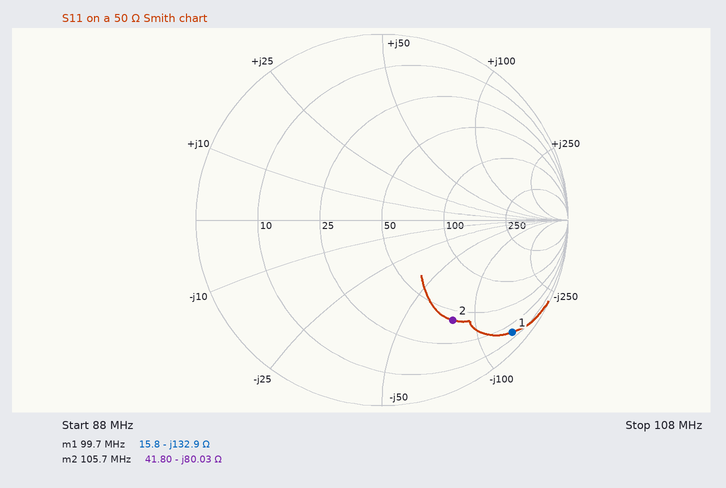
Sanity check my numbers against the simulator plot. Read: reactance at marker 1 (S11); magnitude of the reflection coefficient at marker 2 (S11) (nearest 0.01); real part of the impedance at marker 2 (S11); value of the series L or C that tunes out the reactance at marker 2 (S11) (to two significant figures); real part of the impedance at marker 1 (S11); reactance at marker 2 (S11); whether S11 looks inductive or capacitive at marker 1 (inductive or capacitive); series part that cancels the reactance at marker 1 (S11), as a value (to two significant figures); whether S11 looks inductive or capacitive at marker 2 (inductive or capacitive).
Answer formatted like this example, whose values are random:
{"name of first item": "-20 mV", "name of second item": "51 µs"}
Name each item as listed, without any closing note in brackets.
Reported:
{"reactance at marker 1": "-132.9 Ω", "magnitude of the reflection coefficient at marker 2 (S11)": "0.66", "real part of the impedance at marker 2": "41.80 Ω", "value of the series L or C that tunes out the reactance at marker 2 (S11)": "120 nH", "real part of the impedance at marker 1": "15.8 Ω", "reactance at marker 2": "-80.03 Ω", "whether S11 looks inductive or capacitive at marker 1": "capacitive", "series part that cancels the reactance at marker 1 (S11), as a value": "210 nH", "whether S11 looks inductive or capacitive at marker 2": "capacitive"}
